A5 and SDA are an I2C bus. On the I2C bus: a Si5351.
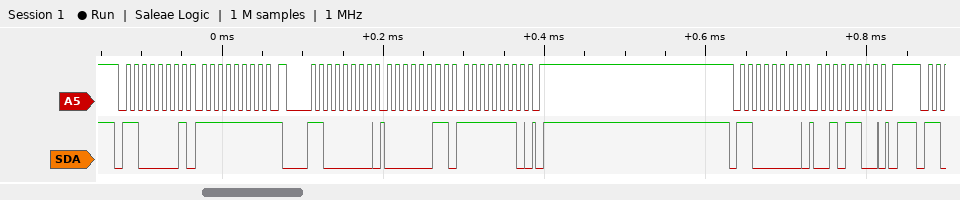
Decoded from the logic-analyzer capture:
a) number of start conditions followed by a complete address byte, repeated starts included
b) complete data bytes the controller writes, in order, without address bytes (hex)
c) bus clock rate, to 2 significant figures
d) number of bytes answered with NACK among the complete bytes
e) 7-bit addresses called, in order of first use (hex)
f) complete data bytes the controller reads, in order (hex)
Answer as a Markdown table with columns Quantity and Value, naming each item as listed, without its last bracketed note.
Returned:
| Quantity | Value |
|---|---|
| number of start conditions followed by a complete address byte, repeated starts included | 3 |
| complete data bytes the controller writes, in order, without address bytes | 03 FE 2C |
| bus clock rate, to 2 significant figures | 100 kHz |
| number of bytes answered with NACK among the complete bytes | 1 |
| 7-bit addresses called, in order of first use | 0x60 |
| complete data bytes the controller reads, in order | FF |
